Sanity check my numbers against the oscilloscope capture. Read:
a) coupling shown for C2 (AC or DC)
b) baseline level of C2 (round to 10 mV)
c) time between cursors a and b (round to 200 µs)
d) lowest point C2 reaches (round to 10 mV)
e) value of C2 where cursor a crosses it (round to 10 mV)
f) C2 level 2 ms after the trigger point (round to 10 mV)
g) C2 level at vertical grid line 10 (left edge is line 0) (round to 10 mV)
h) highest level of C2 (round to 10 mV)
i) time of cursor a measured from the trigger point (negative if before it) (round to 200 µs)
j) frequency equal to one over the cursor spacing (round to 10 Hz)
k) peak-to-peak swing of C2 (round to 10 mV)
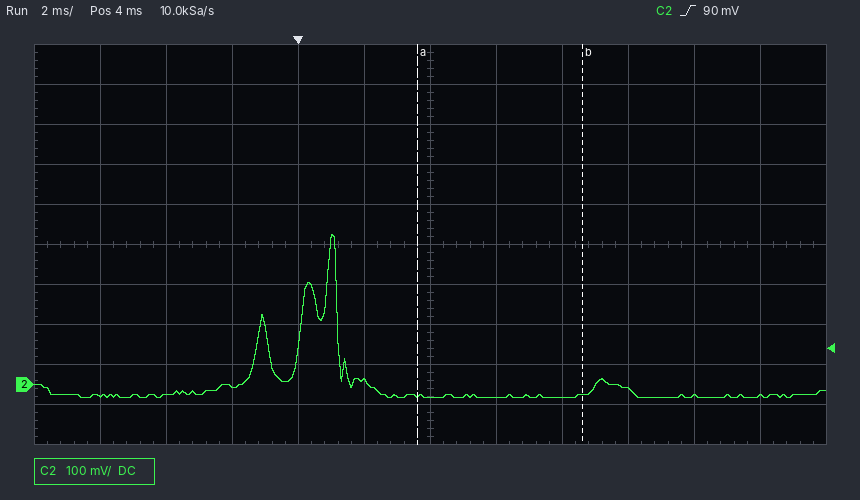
DC
-30 mV
5.0 ms
-30 mV
-30 mV
10 mV
-30 mV
380 mV
+3.6 ms
200 Hz
410 mV
